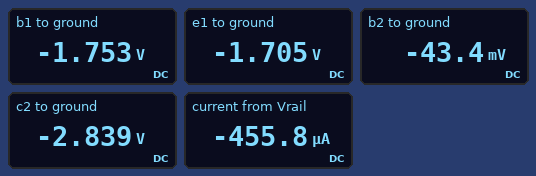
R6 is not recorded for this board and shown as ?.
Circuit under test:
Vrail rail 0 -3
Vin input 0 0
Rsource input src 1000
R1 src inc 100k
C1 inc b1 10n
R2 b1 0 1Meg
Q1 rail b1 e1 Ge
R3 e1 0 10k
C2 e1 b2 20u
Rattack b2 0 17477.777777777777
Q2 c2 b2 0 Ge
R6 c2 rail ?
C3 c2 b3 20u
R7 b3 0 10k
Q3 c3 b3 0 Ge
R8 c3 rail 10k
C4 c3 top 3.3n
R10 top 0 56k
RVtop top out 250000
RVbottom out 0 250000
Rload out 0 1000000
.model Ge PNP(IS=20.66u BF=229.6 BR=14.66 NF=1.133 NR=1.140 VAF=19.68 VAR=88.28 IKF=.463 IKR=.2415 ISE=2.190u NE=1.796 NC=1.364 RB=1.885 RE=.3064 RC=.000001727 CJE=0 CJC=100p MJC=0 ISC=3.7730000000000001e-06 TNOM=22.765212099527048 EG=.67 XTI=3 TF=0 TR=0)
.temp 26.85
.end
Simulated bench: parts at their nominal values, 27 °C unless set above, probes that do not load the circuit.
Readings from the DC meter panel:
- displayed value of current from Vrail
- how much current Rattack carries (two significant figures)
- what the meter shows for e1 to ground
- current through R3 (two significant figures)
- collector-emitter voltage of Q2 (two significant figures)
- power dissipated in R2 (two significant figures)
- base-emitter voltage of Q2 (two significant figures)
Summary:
-455.8 µA
2.5 µA
-1.705 V
170 µA
-2.8 V
3.1 µW
-43 mV
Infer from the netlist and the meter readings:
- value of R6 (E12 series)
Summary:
1 kΩ
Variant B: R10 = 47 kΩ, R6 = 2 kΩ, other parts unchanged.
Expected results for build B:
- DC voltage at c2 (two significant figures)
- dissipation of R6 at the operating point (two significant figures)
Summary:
-2.7 V
51 µW
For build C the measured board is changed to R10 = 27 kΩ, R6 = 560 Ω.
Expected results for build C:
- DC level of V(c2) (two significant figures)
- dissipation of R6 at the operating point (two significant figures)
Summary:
-2.9 V
15 µW
